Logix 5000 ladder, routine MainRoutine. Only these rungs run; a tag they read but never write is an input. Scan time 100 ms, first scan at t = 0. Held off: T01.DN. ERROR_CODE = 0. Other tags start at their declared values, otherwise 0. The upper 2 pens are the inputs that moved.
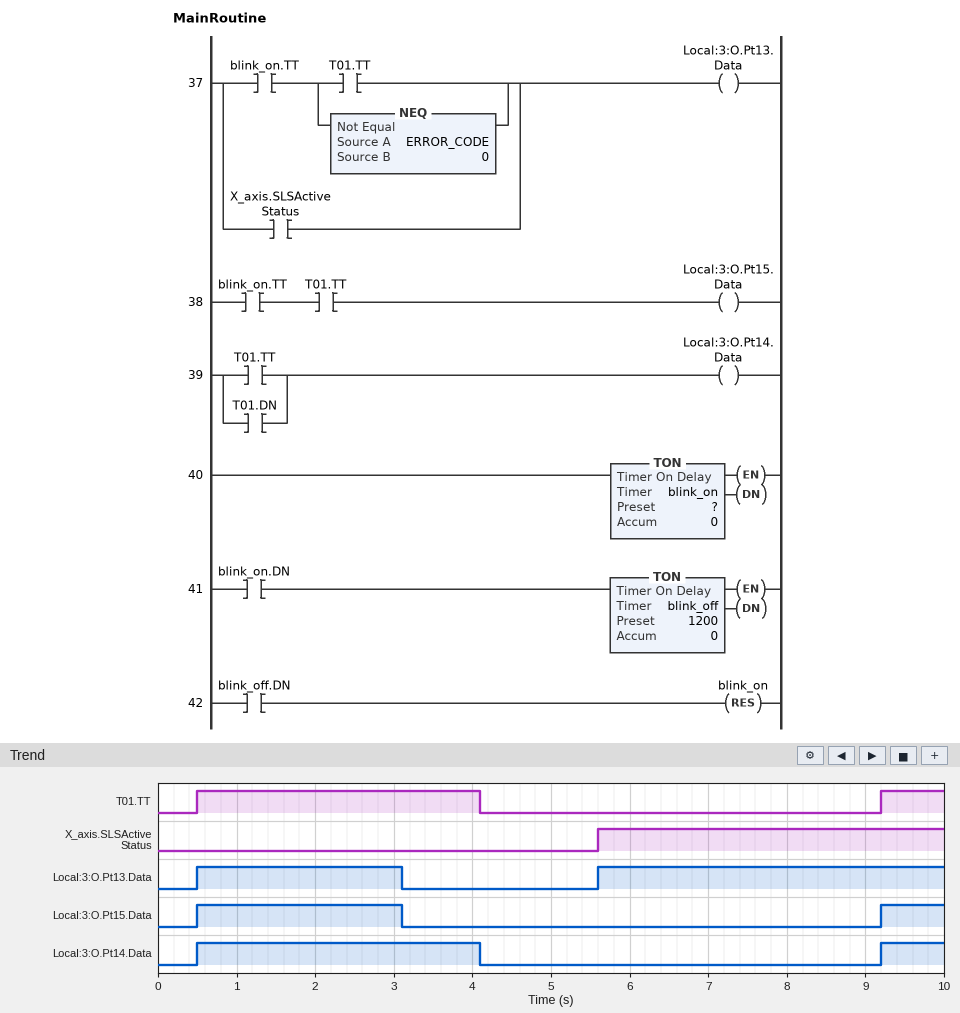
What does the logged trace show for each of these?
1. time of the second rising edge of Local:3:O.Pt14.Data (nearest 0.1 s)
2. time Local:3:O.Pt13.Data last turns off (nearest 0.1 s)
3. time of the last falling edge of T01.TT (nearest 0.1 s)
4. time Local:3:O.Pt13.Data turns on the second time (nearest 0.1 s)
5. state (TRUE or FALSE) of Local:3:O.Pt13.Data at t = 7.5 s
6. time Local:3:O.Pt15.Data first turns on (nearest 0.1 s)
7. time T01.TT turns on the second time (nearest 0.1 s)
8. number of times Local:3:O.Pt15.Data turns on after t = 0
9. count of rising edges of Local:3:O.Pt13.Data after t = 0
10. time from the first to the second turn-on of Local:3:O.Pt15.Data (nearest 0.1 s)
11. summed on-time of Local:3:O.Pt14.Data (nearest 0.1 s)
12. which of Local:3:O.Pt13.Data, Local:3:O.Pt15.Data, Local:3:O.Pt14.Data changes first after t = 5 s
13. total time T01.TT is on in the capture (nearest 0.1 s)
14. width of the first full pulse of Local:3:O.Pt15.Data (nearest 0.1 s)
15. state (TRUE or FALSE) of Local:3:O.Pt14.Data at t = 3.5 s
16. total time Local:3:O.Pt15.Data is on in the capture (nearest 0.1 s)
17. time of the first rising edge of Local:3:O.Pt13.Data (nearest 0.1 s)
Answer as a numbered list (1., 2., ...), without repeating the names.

1. 9.2 s
2. 3.1 s
3. 4.1 s
4. 5.6 s
5. TRUE
6. 0.5 s
7. 9.2 s
8. 2
9. 2
10. 8.7 s
11. 4.4 s
12. Local:3:O.Pt13.Data
13. 4.4 s
14. 2.6 s
15. TRUE
16. 3.4 s
17. 0.5 s
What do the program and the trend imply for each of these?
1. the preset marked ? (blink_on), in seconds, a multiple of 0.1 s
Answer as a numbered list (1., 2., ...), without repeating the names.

1. 3.0 s
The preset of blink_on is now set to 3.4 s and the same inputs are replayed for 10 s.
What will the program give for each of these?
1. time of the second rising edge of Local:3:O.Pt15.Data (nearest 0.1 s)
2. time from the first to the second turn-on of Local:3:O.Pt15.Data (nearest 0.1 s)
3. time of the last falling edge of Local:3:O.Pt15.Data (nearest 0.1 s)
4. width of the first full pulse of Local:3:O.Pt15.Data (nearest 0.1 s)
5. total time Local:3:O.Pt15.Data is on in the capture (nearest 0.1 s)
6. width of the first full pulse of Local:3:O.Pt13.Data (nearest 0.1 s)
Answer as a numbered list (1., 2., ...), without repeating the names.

1. 9.5 s
2. 9.0 s
3. 3.5 s
4. 3.0 s
5. 3.5 s
6. 3.0 s
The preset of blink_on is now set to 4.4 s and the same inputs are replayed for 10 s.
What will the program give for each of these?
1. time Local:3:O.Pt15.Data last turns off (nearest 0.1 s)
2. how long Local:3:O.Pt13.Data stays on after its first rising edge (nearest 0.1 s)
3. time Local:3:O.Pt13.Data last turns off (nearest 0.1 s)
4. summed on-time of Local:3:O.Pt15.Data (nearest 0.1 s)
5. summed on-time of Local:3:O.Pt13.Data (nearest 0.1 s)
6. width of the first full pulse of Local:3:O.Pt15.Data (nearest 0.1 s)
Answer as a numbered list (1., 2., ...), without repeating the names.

1. 4.1 s
2. 3.6 s
3. 4.1 s
4. 4.4 s
5. 8.0 s
6. 3.6 s
